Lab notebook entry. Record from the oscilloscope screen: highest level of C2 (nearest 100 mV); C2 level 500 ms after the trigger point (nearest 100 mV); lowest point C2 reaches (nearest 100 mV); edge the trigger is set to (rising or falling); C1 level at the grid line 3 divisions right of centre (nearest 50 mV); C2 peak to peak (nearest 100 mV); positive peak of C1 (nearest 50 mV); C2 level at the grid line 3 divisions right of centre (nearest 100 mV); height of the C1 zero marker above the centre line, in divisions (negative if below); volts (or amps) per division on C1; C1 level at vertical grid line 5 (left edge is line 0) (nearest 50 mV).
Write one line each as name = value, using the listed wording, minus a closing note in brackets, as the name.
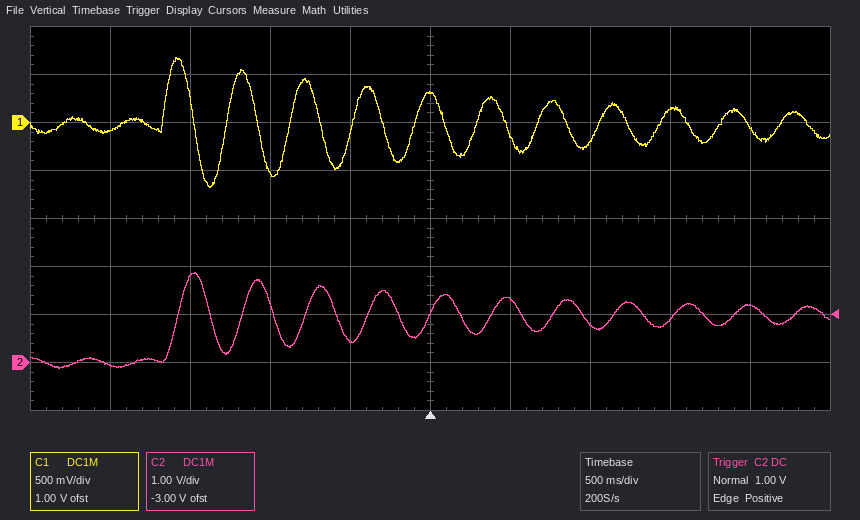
highest level of C2 = 1.9 V
C2 level 500 ms after the trigger point = 1.3 V
lowest point C2 reaches = -100 mV
edge the trigger is set to = rising
C1 level at the grid line 3 divisions right of centre = 150 mV
C2 peak to peak = 2.0 V
positive peak of C1 = 700 mV
C2 level at the grid line 3 divisions right of centre = 900 mV
height of the C1 zero marker above the centre line, in divisions = +2.0 div
volts (or amps) per division on C1 = 500 mV
C1 level at vertical grid line 5 (left edge is line 0) = 300 mV
